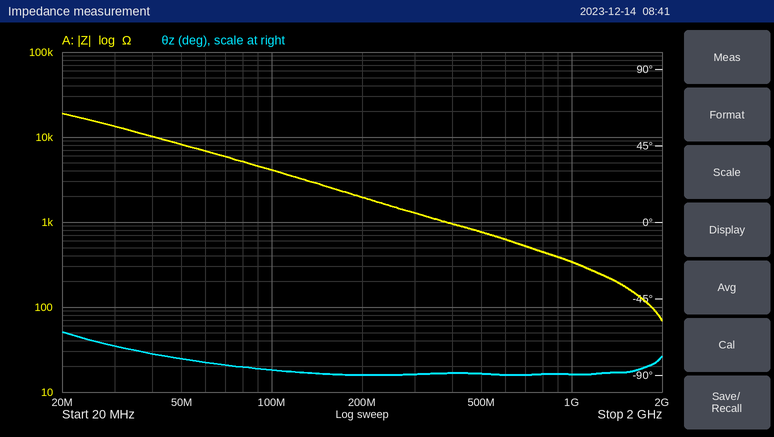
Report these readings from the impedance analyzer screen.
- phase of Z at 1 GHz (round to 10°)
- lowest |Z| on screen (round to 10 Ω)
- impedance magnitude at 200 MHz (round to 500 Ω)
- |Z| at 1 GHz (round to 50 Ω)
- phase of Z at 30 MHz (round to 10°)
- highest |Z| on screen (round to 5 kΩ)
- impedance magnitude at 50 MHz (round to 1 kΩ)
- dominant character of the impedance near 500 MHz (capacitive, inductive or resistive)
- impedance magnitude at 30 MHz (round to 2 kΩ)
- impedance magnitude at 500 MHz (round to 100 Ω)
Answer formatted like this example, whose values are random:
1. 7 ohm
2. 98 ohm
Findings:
1. -90°
2. 70 Ω
3. 2.0 kΩ
4. 350 Ω
5. -70°
6. 20 kΩ
7. 8 kΩ
8. capacitive
9. 14 kΩ
10. 800 Ω
